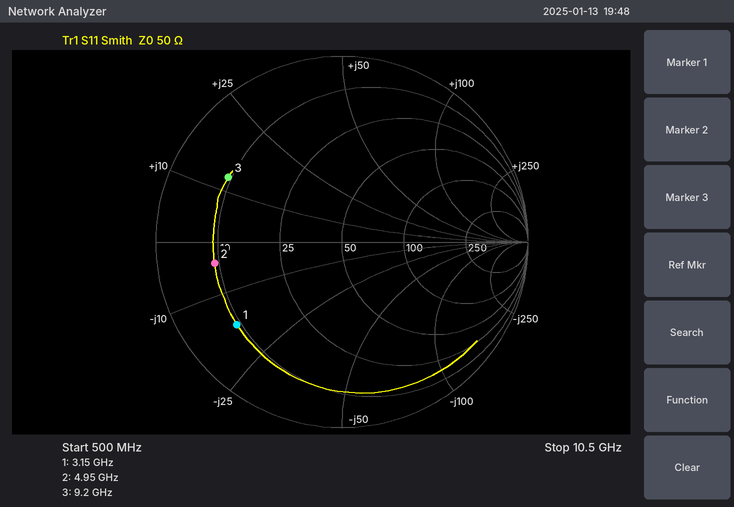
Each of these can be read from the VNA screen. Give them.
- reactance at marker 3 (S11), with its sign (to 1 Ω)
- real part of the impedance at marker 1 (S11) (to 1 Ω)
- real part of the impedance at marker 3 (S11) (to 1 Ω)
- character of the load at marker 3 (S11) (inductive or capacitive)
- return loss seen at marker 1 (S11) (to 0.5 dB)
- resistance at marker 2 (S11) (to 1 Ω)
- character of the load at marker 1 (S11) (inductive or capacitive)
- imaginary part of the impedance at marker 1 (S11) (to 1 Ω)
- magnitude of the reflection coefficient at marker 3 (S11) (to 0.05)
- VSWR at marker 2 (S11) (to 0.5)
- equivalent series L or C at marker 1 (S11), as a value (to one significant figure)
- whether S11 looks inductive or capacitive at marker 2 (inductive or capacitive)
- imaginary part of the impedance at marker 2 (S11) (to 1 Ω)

+13 Ω
9 Ω
9 Ω
inductive
3.0 dB
9 Ω
capacitive
-17 Ω
0.70
5.5
3 pF
capacitive
-4 Ω
